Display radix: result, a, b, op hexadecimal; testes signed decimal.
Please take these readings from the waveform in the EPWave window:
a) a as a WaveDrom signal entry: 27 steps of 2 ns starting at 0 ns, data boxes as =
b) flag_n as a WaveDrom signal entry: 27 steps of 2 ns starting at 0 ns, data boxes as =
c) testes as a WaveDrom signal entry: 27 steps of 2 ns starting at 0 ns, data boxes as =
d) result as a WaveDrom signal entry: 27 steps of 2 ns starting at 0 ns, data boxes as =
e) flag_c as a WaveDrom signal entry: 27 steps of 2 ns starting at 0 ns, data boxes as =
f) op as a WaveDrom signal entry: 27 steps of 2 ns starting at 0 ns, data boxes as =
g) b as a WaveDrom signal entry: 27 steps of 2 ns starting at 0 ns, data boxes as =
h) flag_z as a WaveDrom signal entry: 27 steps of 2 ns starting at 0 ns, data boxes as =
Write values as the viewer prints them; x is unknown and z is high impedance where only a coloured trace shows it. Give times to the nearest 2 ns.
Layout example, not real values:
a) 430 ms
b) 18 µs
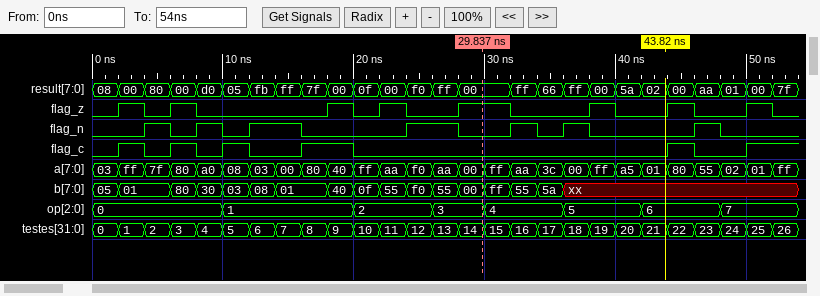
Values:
a) {name: 'a', wave: '===========================', data: '03 ff 7f 80 a0 08 03 00 80 40 ff aa f0 aa 00 ff aa 3c 00 ff a5 01 80 55 02 01 ff'}
b) {name: 'flag_n', wave: '0.10101.0...1.0.1010...10..'}
c) {name: 'testes', wave: '===========================', data: '0 1 2 3 4 5 6 7 8 9 10 11 12 13 14 15 16 17 18 19 20 21 22 23 24 25 26'}
d) {name: 'result', wave: '===============.===========', data: '08 00 80 00 d0 05 fb ff 7f 00 0f 00 f0 ff 00 ff 66 ff 00 5a 02 00 aa 01 00 7f'}
e) {name: 'flag_c', wave: '0101010.1.0...........10.1.'}
f) {name: 'op', wave: '=....=....=..=.=..=..=..=..', data: '0 1 2 3 4 5 6 7'}
g) {name: 'b', wave: '==.=====.=========x........', data: '05 01 80 30 03 08 01 40 0f 55 f0 55 00 ff 55 5a'}
h) {name: 'flag_z', wave: '01010....1010.1.0..10.10.10'}
